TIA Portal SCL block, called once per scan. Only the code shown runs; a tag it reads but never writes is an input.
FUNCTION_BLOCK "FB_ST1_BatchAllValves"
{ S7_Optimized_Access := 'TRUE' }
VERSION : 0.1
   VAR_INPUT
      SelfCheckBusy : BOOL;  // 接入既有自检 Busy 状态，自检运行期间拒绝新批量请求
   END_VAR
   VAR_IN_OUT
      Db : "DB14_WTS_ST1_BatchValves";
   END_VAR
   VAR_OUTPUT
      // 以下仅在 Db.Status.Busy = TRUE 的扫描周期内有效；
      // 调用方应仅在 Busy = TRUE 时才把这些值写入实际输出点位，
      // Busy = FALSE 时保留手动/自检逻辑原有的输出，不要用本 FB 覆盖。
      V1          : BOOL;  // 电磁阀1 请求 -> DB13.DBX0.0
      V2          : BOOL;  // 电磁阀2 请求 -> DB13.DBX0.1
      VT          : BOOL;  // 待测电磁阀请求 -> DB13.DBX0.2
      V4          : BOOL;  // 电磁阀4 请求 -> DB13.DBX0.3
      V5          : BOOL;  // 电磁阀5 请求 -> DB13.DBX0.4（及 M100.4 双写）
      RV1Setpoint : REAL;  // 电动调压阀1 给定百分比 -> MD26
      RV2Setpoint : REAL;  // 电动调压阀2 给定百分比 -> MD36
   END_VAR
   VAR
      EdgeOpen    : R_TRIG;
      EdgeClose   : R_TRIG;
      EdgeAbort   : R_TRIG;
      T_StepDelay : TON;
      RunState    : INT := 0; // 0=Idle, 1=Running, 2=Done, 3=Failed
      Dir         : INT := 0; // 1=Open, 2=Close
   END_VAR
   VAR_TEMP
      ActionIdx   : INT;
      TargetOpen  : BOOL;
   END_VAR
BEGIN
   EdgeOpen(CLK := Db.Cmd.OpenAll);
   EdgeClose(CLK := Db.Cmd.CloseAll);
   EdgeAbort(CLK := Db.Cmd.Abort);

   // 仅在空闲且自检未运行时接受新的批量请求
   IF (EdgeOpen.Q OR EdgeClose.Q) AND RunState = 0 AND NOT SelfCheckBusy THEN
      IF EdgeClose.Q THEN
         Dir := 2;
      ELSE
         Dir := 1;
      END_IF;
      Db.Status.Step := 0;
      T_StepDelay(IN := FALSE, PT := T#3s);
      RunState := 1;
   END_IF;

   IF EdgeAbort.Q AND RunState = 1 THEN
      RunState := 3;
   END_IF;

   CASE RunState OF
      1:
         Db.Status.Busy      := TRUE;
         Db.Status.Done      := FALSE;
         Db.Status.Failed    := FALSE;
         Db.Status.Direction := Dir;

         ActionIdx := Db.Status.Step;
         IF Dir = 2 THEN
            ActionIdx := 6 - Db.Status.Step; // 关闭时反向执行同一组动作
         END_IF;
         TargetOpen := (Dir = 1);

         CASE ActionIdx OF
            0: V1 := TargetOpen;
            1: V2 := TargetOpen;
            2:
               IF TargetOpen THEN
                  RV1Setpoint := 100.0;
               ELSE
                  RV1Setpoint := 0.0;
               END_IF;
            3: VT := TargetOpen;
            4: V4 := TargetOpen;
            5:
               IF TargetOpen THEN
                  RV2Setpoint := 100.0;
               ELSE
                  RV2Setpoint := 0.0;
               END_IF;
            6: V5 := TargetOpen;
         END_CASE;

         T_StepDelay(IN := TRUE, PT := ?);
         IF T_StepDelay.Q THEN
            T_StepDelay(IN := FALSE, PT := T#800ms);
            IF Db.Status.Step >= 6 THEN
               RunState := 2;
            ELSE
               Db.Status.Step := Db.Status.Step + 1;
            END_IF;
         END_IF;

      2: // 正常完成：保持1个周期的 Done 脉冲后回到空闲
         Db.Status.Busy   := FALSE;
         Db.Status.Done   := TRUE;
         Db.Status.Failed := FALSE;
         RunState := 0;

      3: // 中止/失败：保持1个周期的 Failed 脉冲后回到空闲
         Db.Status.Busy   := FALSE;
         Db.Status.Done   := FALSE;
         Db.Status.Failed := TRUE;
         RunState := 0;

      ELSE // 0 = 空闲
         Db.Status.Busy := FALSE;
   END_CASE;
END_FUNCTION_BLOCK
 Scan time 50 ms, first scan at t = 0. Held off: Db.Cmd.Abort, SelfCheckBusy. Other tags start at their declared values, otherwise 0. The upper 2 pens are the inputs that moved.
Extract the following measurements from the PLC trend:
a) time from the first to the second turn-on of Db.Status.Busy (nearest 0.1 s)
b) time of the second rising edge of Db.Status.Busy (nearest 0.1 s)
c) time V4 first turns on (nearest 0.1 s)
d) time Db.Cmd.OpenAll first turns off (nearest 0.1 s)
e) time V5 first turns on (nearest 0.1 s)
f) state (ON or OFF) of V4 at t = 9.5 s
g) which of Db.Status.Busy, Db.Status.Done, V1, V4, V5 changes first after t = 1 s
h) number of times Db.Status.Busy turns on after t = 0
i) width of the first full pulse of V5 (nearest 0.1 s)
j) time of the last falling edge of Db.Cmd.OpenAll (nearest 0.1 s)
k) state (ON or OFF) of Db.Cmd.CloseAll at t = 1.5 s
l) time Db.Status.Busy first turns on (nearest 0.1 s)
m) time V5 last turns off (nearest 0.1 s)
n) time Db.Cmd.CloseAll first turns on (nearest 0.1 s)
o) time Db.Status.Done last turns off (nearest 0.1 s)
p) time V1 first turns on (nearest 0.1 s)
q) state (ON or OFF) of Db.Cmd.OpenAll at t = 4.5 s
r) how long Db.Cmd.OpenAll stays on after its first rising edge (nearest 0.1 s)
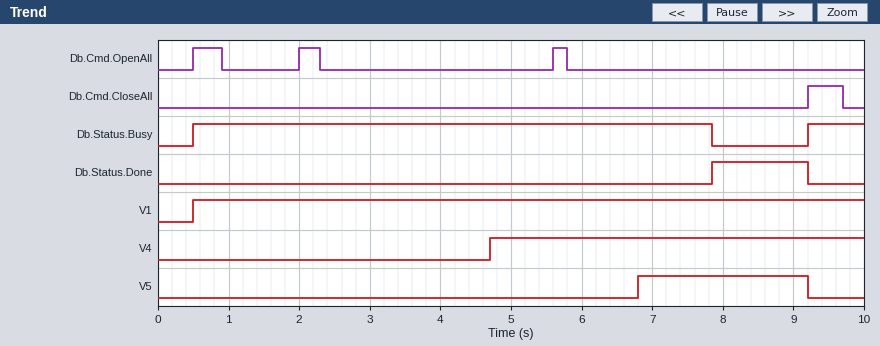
8.7 s
9.2 s
4.7 s
0.9 s
6.8 s
ON
V4
2
2.4 s
5.8 s
OFF
0.5 s
9.2 s
9.2 s
9.2 s
0.5 s
OFF
0.4 s
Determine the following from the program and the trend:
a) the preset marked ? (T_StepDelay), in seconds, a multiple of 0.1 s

1.0 s
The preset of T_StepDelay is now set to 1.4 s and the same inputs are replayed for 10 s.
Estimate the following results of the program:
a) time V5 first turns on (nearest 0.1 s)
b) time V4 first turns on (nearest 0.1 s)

9.2 s
6.3 s
